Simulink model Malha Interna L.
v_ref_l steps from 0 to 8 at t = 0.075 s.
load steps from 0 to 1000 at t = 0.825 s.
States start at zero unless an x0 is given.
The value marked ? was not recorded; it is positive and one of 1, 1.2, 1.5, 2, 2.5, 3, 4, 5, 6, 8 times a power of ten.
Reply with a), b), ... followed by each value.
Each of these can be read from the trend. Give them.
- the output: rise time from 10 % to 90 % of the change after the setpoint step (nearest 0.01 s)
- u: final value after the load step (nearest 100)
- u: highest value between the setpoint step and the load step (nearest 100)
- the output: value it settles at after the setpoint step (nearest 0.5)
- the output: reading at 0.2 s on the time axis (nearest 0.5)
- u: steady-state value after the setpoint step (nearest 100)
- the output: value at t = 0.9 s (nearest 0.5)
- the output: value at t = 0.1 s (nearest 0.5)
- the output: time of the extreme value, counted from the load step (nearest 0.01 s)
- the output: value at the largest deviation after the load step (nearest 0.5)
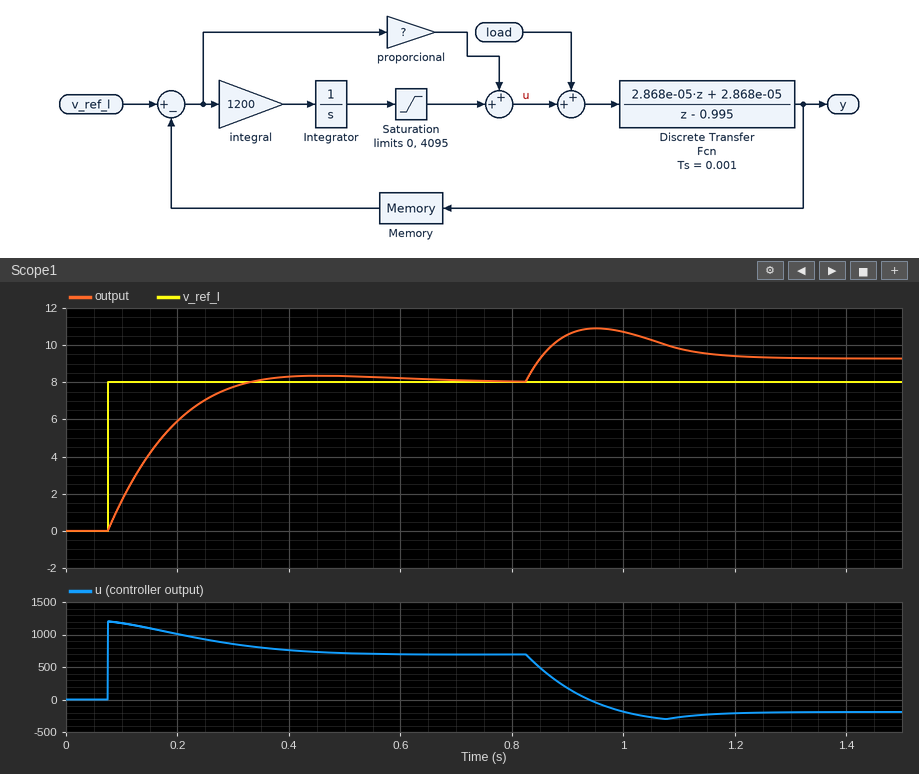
a) 0.17 s
b) -200
c) 1200
d) 8.0
e) 6.0
f) 700
g) 10.5
h) 1.5
i) 0.13 s
j) 11.0
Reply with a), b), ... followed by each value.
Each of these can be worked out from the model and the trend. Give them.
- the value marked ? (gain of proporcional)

a) 150
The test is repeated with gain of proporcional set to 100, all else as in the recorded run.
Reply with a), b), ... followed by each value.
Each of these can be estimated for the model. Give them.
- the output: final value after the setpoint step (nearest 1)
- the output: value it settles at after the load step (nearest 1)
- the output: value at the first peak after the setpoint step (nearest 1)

a) 8
b) 10
c) 9
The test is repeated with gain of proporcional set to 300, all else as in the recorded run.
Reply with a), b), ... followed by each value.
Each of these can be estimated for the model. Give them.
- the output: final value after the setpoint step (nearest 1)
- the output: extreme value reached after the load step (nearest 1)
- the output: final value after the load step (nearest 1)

a) 8
b) 10
c) 9
